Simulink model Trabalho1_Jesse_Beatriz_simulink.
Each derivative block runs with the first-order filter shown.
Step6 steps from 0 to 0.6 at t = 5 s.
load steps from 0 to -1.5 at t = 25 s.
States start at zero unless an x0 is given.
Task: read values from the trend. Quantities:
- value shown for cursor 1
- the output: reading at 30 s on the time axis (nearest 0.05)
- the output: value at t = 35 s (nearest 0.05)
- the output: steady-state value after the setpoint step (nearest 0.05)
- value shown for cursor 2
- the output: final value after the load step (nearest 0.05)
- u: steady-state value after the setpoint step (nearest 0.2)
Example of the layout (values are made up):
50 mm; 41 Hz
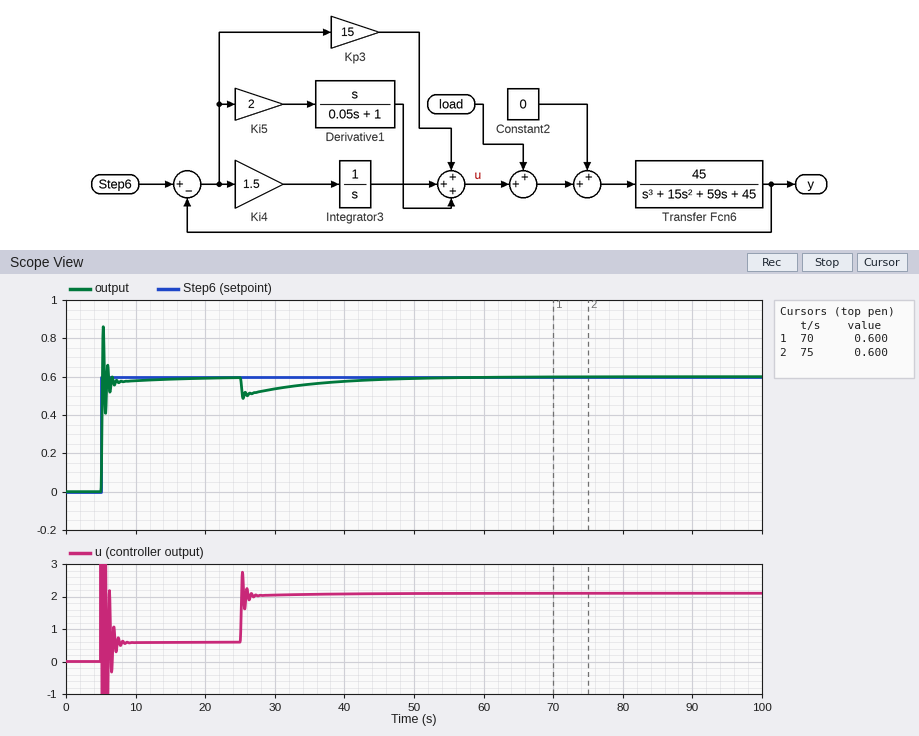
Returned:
0.600; 0.55; 0.55; 0.60; 0.600; 0.60; 0.6
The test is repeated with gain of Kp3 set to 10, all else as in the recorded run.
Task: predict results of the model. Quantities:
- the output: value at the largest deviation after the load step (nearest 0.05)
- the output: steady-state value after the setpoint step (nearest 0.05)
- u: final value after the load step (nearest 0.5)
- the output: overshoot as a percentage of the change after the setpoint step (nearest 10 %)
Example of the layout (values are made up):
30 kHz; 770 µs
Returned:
0.45; 0.60; 2.0; 20 %
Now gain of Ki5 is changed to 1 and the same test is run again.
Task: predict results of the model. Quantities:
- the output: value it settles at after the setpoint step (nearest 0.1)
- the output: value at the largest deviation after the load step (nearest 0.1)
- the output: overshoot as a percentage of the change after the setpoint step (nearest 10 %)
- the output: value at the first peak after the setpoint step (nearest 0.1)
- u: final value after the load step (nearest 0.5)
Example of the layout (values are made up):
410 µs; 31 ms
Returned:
0.6; 0.5; 50 %; 0.9; 2.0
